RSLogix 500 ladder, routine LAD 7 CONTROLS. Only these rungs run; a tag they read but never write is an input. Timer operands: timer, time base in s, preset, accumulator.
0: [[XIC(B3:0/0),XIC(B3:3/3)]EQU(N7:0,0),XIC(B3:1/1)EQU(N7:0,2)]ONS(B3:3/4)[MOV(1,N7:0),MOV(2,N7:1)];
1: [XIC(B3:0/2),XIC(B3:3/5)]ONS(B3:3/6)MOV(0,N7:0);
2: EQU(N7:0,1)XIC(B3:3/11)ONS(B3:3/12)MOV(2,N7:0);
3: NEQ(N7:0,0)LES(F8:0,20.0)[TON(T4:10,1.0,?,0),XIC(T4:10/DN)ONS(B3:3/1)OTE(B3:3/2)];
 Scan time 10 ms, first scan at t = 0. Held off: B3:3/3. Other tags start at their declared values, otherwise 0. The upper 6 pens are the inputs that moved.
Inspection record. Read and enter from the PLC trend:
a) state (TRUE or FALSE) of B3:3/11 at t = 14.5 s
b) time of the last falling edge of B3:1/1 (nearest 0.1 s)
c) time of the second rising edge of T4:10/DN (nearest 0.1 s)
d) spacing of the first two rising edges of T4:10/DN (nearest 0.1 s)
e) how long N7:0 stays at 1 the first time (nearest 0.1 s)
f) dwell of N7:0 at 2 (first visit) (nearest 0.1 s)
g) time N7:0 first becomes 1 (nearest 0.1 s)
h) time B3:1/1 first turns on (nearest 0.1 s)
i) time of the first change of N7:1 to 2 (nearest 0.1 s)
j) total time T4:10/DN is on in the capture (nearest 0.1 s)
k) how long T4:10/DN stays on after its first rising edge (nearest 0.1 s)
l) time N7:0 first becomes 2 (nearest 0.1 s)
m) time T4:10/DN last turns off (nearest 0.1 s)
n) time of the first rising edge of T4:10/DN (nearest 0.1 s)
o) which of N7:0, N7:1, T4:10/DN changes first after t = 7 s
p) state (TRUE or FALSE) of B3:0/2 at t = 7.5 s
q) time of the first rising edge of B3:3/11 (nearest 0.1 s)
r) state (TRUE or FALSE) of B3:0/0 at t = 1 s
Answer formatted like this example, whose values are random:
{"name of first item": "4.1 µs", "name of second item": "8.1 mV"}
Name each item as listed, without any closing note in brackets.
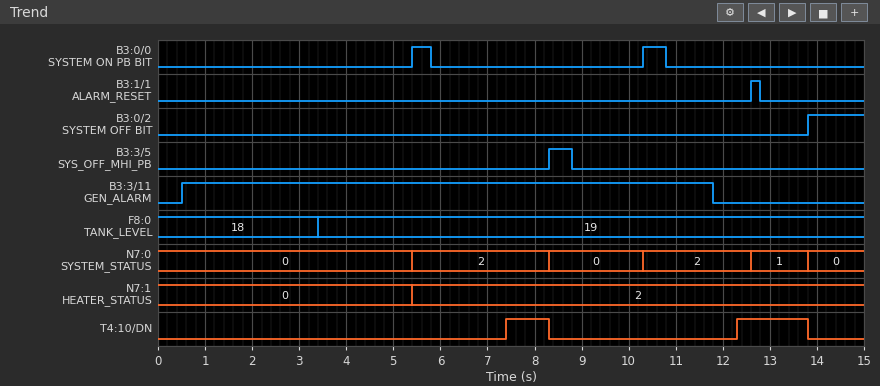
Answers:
{"state (TRUE or FALSE) of B3:3/11 at t = 14.5 s": "FALSE", "time of the last falling edge of B3:1/1": "12.8 s", "time of the second rising edge of T4:10/DN": "12.3 s", "spacing of the first two rising edges of T4:10/DN": "4.9 s", "how long N7:0 stays at 1 the first time": "1.2 s", "dwell of N7:0 at 2 (first visit)": "2.9 s", "time N7:0 first becomes 1": "12.6 s", "time B3:1/1 first turns on": "12.6 s", "time of the first change of N7:1 to 2": "5.4 s", "total time T4:10/DN is on in the capture": "2.4 s", "how long T4:10/DN stays on after its first rising edge": "0.9 s", "time N7:0 first becomes 2": "5.4 s", "time T4:10/DN last turns off": "13.8 s", "time of the first rising edge of T4:10/DN": "7.4 s", "which of N7:0, N7:1, T4:10/DN changes first after t = 7 s": "T4:10/DN", "state (TRUE or FALSE) of B3:0/2 at t = 7.5 s": "FALSE", "time of the first rising edge of B3:3/11": "0.5 s", "state (TRUE or FALSE) of B3:0/0 at t = 1 s": "FALSE"}
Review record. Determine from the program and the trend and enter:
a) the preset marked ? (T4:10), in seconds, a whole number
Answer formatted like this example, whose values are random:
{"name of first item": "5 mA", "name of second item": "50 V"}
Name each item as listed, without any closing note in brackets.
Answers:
{"the preset marked ? (T4:10), in seconds, a whole number": "2 s"}
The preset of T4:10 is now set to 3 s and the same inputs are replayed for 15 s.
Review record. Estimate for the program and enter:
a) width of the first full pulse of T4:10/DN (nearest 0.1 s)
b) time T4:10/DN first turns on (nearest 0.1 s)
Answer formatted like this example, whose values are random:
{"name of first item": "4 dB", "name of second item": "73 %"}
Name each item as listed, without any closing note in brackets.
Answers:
{"width of the first full pulse of T4:10/DN": "0.5 s", "time T4:10/DN first turns on": "13.3 s"}
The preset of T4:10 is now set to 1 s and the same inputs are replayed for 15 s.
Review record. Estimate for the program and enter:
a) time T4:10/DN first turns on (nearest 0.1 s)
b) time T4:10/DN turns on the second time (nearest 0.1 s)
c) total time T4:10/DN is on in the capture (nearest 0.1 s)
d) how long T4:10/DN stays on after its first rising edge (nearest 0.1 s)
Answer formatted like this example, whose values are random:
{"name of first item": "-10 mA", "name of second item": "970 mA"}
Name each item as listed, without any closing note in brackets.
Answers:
{"time T4:10/DN first turns on": "6.4 s", "time T4:10/DN turns on the second time": "11.3 s", "total time T4:10/DN is on in the capture": "4.4 s", "how long T4:10/DN stays on after its first rising edge": "1.9 s"}
